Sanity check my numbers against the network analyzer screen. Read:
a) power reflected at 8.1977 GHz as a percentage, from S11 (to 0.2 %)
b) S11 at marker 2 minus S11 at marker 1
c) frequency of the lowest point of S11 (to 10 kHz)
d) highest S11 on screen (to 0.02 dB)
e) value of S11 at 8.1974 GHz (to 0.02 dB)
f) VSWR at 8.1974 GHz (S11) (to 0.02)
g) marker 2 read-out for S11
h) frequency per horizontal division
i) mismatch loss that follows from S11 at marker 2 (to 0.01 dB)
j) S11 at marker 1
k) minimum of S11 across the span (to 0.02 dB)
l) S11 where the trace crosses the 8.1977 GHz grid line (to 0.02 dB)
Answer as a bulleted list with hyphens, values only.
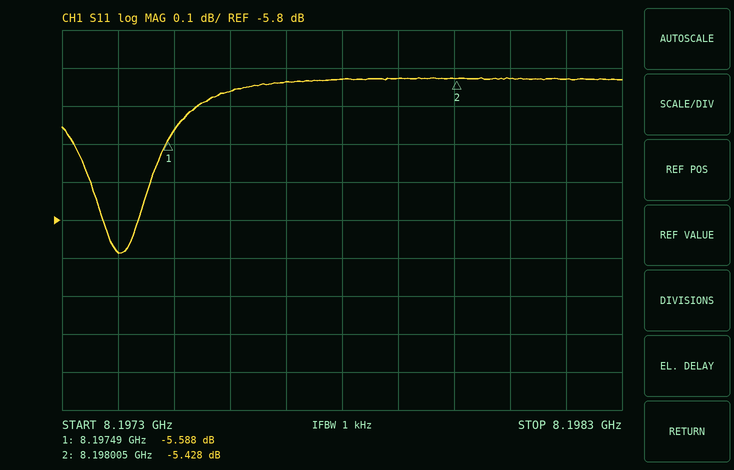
- 28.6 %
- 0.160 dB
- 8.19740 GHz
- -5.42 dB
- -5.88 dB
- 3.06
- -5.428 dB
- 100 kHz
- 1.47 dB
- -5.588 dB
- -5.88 dB
- -5.44 dB
